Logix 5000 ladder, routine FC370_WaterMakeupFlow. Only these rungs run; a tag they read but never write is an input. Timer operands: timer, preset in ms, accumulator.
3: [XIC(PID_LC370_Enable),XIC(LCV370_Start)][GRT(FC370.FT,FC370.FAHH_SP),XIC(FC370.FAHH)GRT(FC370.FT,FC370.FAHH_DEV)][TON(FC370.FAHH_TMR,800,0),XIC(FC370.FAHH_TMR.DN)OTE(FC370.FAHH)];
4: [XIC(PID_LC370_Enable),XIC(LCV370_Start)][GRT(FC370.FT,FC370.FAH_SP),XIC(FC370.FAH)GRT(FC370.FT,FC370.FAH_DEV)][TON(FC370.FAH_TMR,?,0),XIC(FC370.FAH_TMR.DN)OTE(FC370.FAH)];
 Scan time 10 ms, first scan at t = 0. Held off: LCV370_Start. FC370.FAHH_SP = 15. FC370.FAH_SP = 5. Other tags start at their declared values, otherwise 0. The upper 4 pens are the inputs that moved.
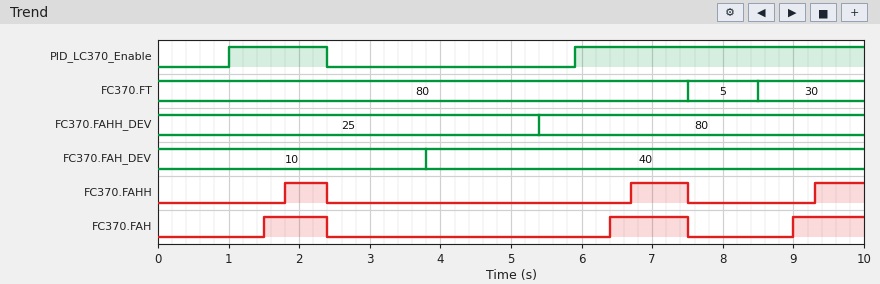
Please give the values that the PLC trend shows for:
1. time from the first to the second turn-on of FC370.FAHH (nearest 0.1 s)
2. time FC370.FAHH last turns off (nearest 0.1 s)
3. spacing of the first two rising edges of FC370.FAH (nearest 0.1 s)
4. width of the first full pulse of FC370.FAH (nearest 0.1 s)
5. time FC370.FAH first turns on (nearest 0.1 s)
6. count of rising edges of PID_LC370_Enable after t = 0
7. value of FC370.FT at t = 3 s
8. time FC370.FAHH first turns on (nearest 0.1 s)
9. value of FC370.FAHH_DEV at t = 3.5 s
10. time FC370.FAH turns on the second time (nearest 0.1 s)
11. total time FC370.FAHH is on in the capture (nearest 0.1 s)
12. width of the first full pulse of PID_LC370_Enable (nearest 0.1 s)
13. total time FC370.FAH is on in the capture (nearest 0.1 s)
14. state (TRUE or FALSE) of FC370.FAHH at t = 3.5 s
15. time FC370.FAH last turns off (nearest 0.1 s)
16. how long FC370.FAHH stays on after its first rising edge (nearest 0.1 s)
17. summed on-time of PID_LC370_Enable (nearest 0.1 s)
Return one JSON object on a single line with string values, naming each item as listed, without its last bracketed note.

{"time from the first to the second turn-on of FC370.FAHH": "4.9 s", "time FC370.FAHH last turns off": "7.5 s", "spacing of the first two rising edges of FC370.FAH": "4.9 s", "width of the first full pulse of FC370.FAH": "0.9 s", "time FC370.FAH first turns on": "1.5 s", "count of rising edges of PID_LC370_Enable after t = 0": "2", "value of FC370.FT at t = 3 s": "80", "time FC370.FAHH first turns on": "1.8 s", "value of FC370.FAHH_DEV at t = 3.5 s": "25", "time FC370.FAH turns on the second time": "6.4 s", "total time FC370.FAHH is on in the capture": "2.1 s", "width of the first full pulse of PID_LC370_Enable": "1.4 s", "total time FC370.FAH is on in the capture": "3.0 s", "state (TRUE or FALSE) of FC370.FAHH at t = 3.5 s": "FALSE", "time FC370.FAH last turns off": "7.5 s", "how long FC370.FAHH stays on after its first rising edge": "0.6 s", "summed on-time of PID_LC370_Enable": "5.5 s"}
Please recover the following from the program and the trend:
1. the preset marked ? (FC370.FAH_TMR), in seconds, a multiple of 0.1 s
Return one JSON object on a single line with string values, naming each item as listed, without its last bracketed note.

{"the preset marked ? (FC370.FAH_TMR), in seconds, a multiple of 0.1 s": "0.5 s"}
